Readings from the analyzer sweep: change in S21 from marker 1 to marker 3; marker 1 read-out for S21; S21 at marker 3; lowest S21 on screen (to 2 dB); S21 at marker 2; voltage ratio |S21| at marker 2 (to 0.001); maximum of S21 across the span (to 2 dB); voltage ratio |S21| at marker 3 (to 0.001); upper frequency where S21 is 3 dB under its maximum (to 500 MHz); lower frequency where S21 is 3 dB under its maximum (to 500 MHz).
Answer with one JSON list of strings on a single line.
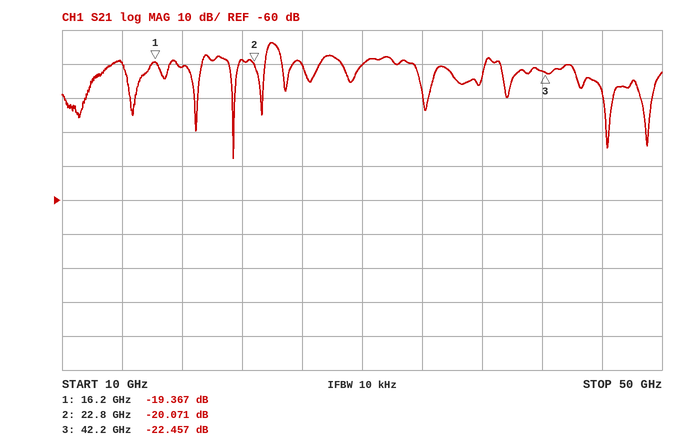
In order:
["-3.090 dB", "-19.367 dB", "-22.457 dB", "-48 dB", "-20.071 dB", "0.099", "-14 dB", "0.075", "24.5 GHz", "23.5 GHz"]
